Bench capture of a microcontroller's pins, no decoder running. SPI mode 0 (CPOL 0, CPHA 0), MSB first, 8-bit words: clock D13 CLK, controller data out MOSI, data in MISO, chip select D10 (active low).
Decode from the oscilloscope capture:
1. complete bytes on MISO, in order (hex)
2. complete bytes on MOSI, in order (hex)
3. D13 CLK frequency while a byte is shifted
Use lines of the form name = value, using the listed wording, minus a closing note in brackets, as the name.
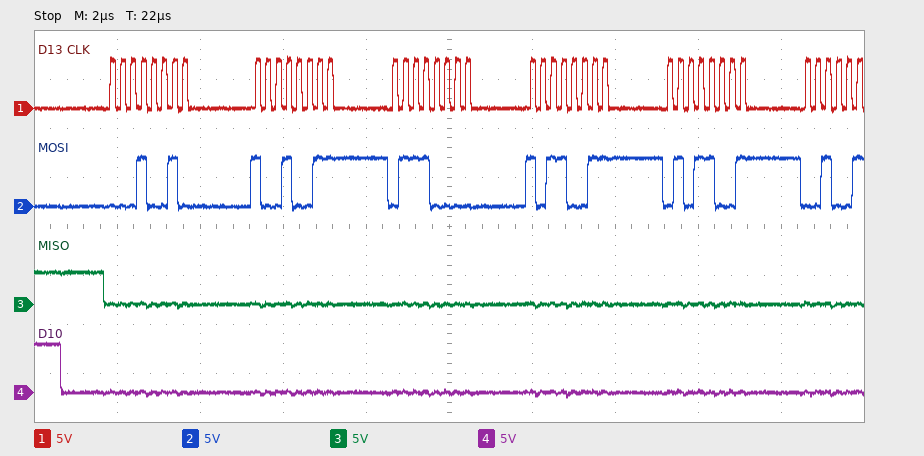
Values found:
complete bytes on MISO, in order = 00 00 00 00 00
complete bytes on MOSI, in order = 12 93 70 B3 59
D13 CLK frequency while a byte is shifted = 4 MHz
